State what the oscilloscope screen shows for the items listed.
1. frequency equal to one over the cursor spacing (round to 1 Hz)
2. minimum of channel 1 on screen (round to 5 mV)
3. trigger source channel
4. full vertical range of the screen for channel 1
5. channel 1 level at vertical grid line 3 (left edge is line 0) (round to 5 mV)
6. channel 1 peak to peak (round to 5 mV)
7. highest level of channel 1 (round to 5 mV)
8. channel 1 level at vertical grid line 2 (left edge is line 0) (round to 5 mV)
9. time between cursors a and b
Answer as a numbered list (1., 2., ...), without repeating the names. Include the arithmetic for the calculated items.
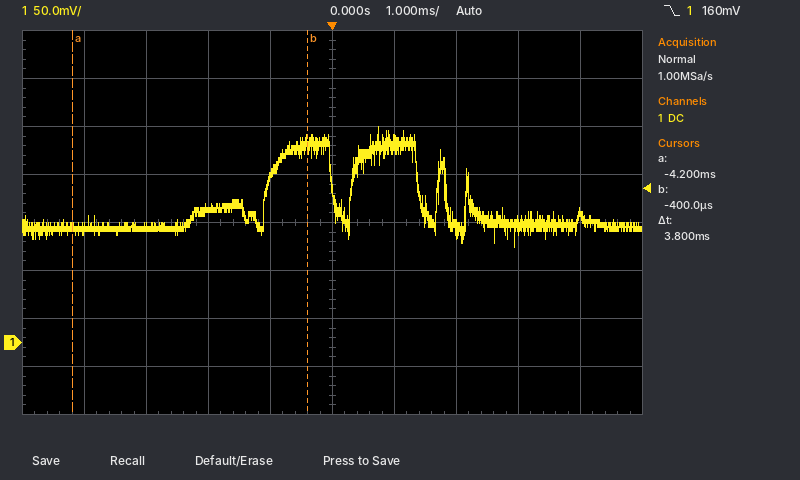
1. 1 / 3.8 ms ≈ 263 Hz
2. 100 mV
3. channel 1
4. 400 mV
5. 140 mV
6. 225 mV − (100 mV) = 125 mV
7. 225 mV
8. 120 mV
9. 3.8 ms
